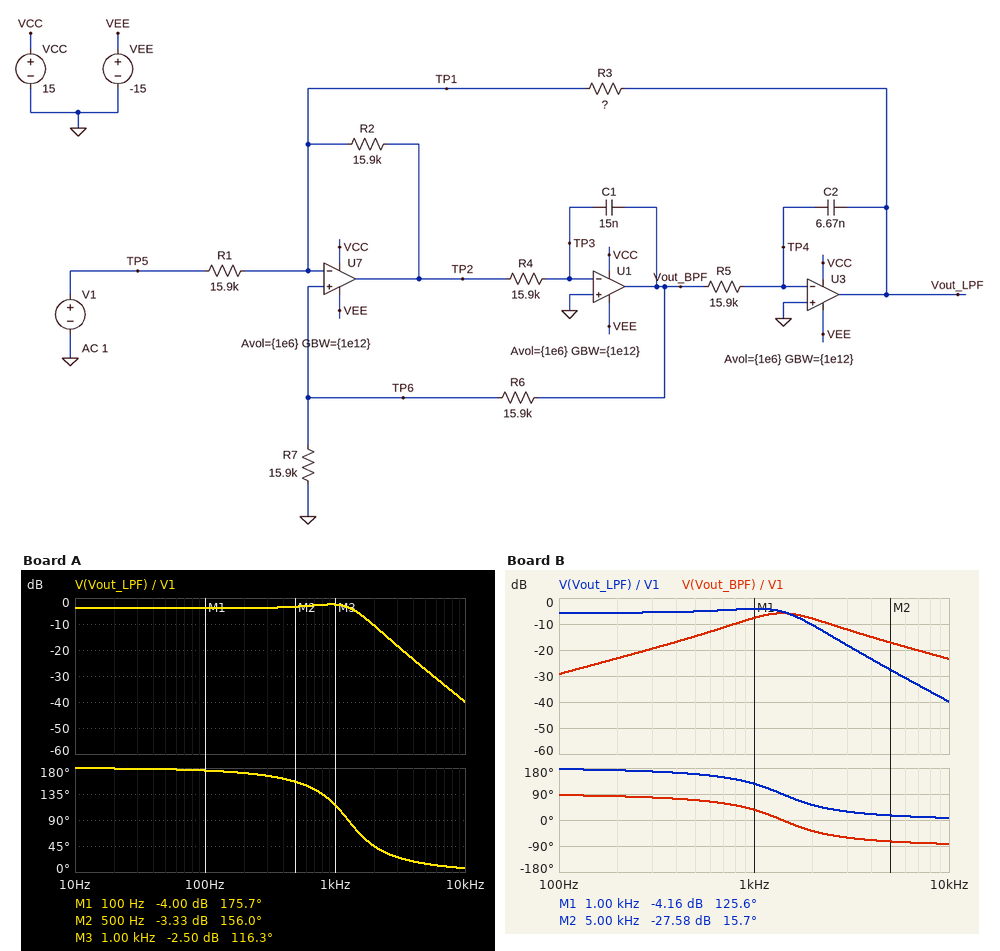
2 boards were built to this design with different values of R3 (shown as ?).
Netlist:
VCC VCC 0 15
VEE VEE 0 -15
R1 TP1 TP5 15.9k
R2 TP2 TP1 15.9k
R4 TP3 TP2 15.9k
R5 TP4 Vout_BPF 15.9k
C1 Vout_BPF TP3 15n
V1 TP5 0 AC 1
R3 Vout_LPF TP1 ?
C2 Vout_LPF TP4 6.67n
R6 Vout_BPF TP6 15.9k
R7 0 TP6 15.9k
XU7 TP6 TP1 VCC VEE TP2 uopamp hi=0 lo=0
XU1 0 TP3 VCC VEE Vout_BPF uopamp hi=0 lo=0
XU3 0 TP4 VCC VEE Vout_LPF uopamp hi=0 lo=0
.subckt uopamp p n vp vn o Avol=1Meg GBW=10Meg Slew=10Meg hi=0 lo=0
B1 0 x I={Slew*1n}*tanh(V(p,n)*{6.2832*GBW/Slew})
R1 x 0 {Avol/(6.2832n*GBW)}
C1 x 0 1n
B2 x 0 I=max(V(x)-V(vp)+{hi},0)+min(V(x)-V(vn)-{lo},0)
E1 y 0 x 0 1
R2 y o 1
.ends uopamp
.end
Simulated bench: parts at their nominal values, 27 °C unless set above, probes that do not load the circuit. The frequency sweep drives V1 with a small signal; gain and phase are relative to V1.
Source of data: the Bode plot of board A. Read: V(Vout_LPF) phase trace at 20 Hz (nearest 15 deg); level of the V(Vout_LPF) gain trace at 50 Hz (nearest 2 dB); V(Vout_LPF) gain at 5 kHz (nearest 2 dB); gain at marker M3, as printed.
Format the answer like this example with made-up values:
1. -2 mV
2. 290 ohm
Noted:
1. 180 deg
2. -4 dB
3. -28 dB
4. -2.50 dB
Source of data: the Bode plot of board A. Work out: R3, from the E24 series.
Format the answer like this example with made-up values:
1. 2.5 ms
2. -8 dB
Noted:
1. 10 kΩ
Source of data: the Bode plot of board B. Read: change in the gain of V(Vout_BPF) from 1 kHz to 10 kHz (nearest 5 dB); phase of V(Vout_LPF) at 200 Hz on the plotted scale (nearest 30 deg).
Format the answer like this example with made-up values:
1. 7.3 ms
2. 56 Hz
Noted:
1. -15 dB
2. 180 deg
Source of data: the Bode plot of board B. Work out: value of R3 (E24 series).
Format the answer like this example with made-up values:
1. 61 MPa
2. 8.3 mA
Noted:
1. 8.2 kΩ
